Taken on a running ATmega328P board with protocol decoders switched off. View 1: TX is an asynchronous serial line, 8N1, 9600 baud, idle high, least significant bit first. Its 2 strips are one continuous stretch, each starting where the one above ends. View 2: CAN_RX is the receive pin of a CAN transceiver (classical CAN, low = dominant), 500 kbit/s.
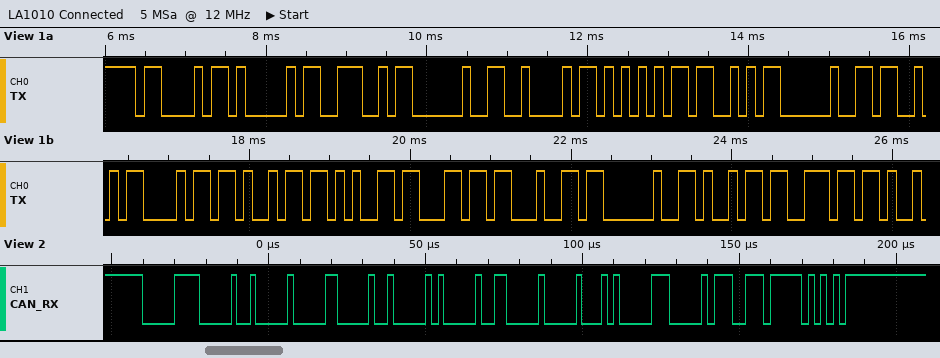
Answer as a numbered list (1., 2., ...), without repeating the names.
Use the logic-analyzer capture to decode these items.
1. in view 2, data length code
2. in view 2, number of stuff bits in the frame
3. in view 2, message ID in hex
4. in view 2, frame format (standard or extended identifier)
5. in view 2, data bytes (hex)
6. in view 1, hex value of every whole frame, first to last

1. 8
2. 12
3. 0x070
4. standard
5. 01 01 02 03 00 05 06 07
6. 43 41 4E 20 42 55 53 20 53 68 69 65 6C 64 20 69 6E
